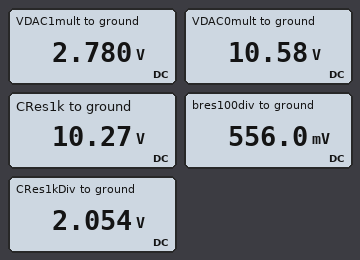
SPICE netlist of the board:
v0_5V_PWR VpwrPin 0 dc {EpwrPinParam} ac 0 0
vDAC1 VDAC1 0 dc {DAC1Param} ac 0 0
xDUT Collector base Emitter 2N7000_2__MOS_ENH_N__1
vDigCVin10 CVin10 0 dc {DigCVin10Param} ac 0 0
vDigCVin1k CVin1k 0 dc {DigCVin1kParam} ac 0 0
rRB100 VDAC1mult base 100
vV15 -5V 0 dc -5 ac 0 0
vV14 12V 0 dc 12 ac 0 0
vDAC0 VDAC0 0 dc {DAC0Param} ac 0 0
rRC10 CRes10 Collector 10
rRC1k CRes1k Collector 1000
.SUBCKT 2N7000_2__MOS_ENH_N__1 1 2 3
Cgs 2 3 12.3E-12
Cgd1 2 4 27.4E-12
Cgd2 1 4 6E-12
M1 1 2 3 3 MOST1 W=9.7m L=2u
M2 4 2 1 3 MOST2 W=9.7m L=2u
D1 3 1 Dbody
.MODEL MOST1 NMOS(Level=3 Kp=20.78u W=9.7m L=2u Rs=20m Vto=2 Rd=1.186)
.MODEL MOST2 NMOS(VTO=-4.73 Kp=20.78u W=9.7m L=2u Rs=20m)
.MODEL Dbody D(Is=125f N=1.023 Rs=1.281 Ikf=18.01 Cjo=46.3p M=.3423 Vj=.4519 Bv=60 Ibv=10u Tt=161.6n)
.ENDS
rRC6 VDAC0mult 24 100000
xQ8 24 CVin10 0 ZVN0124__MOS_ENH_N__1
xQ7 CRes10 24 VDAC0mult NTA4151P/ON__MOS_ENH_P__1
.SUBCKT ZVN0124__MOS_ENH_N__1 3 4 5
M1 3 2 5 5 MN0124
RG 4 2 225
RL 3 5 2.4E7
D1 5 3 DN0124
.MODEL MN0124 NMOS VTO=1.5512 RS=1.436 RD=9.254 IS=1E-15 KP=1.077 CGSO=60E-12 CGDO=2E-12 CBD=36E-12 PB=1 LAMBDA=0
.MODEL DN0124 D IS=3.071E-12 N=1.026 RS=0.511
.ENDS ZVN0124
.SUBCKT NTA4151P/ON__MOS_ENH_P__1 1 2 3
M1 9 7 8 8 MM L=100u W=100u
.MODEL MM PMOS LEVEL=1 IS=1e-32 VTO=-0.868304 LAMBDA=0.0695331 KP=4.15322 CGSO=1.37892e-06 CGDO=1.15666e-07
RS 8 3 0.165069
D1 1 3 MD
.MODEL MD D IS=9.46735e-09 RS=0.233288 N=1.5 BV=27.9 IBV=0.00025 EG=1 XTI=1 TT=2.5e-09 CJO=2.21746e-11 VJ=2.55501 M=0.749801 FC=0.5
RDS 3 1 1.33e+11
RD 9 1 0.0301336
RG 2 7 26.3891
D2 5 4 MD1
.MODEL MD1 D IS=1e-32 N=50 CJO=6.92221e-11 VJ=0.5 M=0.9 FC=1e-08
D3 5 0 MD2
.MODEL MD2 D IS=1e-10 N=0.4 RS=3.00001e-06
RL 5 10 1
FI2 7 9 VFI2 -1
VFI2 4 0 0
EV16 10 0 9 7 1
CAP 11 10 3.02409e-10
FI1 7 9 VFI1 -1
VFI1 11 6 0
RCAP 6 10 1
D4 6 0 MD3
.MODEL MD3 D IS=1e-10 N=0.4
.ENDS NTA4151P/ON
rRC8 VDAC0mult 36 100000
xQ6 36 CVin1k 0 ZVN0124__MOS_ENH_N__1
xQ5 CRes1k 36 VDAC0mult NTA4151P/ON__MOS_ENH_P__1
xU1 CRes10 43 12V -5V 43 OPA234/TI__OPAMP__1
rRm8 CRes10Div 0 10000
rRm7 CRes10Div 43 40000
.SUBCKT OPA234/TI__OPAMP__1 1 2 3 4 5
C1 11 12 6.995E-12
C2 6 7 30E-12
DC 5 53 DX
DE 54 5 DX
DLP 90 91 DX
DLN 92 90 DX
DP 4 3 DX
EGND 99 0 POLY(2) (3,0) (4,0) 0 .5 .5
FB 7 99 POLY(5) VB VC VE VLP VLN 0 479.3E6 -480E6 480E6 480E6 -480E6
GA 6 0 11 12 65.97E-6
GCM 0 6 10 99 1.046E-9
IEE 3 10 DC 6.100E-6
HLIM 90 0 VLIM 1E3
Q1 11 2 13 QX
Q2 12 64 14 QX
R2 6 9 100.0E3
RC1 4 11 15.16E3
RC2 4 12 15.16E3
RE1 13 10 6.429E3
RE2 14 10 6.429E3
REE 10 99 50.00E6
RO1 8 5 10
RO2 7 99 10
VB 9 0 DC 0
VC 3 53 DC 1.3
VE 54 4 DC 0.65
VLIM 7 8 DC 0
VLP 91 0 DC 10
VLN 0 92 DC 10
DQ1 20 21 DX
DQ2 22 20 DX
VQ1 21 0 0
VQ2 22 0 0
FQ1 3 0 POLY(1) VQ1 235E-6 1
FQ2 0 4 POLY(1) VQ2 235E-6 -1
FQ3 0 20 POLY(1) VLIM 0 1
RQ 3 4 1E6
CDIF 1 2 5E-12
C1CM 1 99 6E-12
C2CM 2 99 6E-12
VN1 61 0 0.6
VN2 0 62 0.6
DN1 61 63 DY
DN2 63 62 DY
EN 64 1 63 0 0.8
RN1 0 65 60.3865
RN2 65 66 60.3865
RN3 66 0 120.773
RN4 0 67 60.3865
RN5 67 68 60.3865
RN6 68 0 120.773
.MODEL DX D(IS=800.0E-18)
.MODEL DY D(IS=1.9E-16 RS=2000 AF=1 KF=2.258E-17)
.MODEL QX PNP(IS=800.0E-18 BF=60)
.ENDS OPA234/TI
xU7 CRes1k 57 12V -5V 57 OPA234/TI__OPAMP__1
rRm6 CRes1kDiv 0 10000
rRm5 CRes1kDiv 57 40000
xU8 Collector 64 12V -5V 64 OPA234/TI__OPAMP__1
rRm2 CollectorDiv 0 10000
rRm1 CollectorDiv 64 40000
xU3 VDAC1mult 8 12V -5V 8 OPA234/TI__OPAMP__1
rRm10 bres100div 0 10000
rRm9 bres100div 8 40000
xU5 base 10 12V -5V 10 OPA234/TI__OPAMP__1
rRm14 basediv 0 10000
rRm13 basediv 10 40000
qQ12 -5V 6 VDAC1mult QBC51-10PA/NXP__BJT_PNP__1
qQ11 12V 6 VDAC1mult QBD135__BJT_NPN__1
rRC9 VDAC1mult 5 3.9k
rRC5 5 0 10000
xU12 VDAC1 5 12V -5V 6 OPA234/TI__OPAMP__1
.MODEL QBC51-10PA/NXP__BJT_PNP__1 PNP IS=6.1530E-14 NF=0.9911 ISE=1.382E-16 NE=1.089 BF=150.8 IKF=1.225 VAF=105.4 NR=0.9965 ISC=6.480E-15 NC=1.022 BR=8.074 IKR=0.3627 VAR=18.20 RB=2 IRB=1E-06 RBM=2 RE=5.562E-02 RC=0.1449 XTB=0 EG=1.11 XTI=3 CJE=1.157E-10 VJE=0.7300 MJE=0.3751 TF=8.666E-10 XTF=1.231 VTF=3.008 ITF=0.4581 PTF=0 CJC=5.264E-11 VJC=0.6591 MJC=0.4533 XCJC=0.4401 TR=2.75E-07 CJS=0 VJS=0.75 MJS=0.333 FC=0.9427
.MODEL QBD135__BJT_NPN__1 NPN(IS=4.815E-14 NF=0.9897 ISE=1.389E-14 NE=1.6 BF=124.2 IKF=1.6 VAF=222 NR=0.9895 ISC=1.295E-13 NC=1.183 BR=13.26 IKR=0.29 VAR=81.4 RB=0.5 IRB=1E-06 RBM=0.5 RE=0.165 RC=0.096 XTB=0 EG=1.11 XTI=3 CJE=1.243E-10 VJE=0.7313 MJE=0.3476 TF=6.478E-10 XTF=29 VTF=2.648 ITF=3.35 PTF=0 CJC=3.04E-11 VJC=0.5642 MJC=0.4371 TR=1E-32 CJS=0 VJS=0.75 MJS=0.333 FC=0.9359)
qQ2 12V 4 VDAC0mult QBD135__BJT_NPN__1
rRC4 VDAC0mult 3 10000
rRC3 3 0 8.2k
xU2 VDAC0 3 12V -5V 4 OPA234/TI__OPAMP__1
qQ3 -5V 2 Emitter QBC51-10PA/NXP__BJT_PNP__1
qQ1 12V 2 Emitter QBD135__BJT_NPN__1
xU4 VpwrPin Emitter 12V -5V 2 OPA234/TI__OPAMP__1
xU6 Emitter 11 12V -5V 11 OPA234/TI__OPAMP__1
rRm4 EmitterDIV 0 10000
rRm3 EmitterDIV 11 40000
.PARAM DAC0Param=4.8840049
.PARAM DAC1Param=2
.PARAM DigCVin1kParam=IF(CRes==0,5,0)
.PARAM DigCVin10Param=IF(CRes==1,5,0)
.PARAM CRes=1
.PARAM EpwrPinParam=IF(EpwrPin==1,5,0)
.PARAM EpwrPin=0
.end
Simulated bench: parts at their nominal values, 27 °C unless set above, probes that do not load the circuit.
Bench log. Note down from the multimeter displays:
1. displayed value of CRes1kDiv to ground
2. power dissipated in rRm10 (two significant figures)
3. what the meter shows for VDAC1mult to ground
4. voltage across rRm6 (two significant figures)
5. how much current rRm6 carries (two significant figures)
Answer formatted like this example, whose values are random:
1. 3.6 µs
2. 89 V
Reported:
1. 2.054 V
2. 31 µW
3. 2.780 V
4. 2.1 V
5. 210 µA
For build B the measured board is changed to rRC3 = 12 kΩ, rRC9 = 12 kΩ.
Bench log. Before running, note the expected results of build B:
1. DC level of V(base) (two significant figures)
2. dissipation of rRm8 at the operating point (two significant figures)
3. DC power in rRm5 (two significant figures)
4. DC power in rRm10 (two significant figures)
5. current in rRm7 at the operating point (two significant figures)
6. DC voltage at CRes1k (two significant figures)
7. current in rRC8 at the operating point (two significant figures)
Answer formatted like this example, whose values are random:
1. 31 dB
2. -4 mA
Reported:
1. 4.4 V
2. 320 µW
3. 580 µW
4. 77 µW
5. 180 µA
6. 6.0 V
7. 370 nA
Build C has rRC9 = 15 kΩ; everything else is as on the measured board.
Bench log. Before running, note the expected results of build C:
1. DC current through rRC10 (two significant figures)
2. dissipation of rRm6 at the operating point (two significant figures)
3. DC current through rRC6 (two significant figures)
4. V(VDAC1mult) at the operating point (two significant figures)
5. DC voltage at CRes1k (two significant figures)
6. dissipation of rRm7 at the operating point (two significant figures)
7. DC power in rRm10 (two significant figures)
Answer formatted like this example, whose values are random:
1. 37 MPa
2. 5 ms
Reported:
1. 450 mA
2. 140 µW
3. 100 µA
4. 5.0 V
5. 5.8 V
6. 1.7 mW
7. 100 µW
